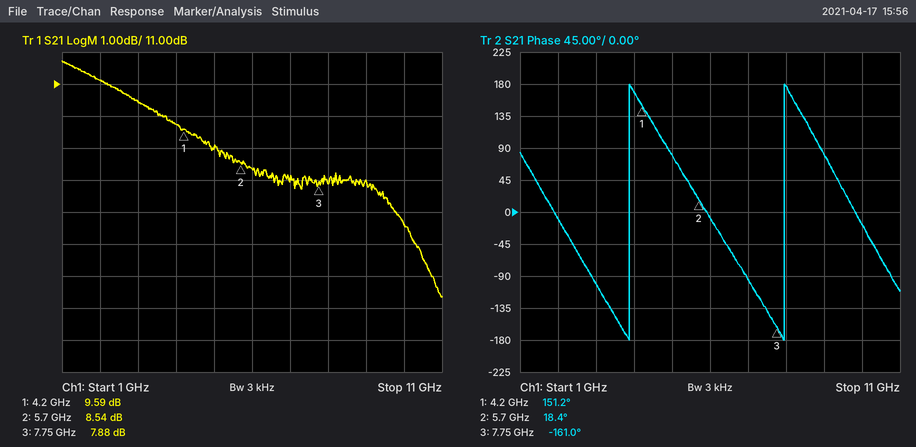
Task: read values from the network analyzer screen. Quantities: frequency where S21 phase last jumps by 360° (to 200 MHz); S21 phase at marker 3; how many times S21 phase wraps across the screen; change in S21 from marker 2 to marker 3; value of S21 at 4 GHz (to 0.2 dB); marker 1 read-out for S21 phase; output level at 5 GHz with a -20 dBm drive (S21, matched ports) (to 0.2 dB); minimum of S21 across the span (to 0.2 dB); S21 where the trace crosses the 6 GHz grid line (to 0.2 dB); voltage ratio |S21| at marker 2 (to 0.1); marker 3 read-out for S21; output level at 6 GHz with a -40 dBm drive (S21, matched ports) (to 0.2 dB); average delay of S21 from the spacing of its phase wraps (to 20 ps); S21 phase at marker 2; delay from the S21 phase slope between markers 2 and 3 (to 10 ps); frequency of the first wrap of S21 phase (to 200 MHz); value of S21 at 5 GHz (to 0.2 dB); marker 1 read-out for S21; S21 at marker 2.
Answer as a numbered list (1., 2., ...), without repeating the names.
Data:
1. 8.0 GHz
2. -161.0°
3. 2
4. -0.66 dB
5. 9.8 dB
6. 151.2°
7. -11.0 dBm
8. 4.4 dB
9. 8.4 dB
10. 2.7
11. 7.88 dB
12. -31.6 dBm
13. 240 ps
14. 18.4°
15. 240 ps
16. 3.8 GHz
17. 9.0 dB
18. 9.59 dB
19. 8.54 dB
